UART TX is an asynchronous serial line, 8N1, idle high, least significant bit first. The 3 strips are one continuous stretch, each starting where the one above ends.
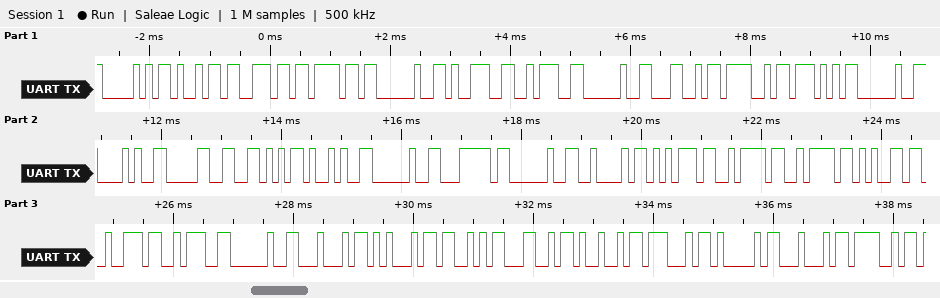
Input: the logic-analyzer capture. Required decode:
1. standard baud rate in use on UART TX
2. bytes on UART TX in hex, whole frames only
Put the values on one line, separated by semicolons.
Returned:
9600 baud; 0x50 0x69 0x6E 0x6F 0x20 0x39 0x3A 0x20 0x4C 0x4F 0x57 0x20 0x28 0x30 0x56 0x29 0x20 0x7C 0x20 0x42 0x75 0x7A 0x7A 0x65 0x72 0x3A 0x20 0x44 0x45 0x53 0x4C 0x49 0x47 0x41 0x44 0x4F
